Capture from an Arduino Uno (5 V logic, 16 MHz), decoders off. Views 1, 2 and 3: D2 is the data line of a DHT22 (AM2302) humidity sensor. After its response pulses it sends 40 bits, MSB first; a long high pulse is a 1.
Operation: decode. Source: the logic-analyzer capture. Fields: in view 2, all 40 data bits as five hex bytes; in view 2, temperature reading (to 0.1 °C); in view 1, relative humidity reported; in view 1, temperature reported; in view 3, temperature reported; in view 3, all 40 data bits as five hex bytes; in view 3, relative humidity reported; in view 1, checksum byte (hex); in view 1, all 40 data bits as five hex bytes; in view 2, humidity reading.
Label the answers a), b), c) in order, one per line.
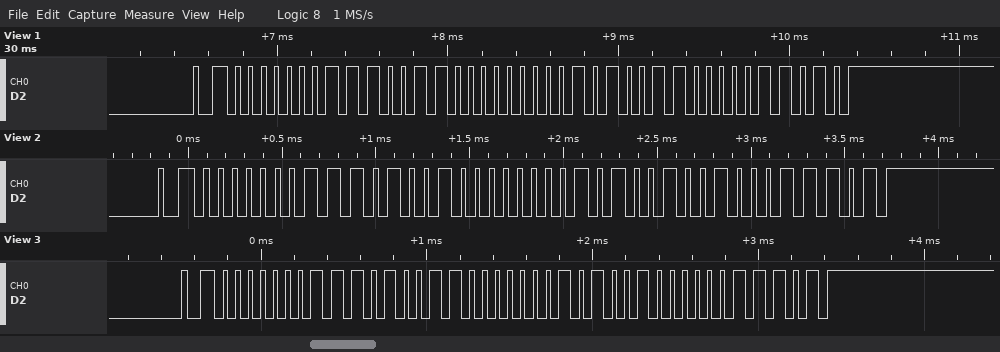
a) 01 D2 01 49 1D
b) 32.9 °C
c) 46.0 %
d) 33.2 °C
e) 32.8 °C
f) 01 D3 01 48 1D
g) 46.7 %
h) 0x1A
i) 01 CC 01 4C 1A
j) 46.6 %
